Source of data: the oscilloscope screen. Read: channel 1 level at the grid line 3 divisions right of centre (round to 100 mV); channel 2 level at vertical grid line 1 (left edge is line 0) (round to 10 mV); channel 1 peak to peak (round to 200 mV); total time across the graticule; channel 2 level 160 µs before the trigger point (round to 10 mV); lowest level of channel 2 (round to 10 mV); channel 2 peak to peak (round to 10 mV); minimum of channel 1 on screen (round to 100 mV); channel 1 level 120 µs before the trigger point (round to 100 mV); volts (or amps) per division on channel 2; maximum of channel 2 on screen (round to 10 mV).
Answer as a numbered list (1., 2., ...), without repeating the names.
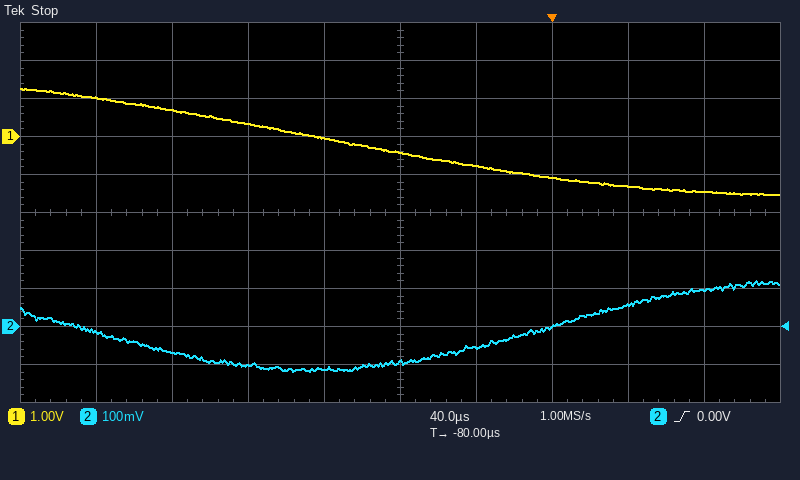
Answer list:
1. -1.3 V
2. -10 mV
3. 2.8 V
4. 400 µs
5. -100 mV
6. -120 mV
7. 240 mV
8. -1.5 V
9. 0.0 V
10. 100 mV
11. 120 mV
